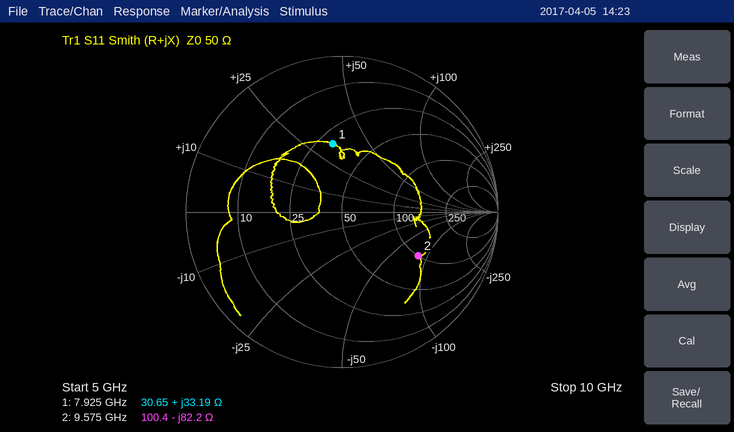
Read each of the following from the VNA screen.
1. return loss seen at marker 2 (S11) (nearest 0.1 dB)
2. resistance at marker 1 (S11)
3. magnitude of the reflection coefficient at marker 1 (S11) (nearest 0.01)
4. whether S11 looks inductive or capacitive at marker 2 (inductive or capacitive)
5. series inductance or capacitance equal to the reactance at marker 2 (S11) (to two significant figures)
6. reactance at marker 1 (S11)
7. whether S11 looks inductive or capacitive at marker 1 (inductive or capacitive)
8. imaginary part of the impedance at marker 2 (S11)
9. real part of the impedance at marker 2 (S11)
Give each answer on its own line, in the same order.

5.0 dB
30.65 Ω
0.44
capacitive
200 fF
+33.19 Ω
inductive
-82.2 Ω
100.4 Ω
